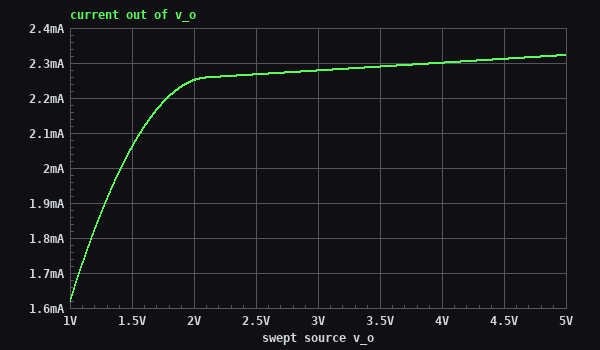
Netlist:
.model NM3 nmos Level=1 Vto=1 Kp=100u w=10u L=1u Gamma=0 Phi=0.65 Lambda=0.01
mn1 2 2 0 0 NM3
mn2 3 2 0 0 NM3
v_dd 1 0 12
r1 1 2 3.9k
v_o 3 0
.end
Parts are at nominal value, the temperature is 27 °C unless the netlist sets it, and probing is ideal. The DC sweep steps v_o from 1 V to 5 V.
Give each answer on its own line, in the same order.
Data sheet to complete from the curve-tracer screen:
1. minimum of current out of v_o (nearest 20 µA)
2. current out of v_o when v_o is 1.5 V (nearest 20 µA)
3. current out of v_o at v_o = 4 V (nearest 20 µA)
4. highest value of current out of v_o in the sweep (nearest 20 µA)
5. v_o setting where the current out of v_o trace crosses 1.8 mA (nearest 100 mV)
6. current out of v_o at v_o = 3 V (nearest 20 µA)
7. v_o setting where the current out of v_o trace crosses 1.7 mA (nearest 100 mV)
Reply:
1.62 mA
2.06 mA
2.30 mA
2.32 mA
1.2 V
2.28 mA
1.1 V
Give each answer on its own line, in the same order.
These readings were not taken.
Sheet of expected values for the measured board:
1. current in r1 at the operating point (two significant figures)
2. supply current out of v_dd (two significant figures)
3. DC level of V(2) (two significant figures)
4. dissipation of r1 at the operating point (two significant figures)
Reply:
2.3 mA
2.3 mA
3.1 V
20 mW
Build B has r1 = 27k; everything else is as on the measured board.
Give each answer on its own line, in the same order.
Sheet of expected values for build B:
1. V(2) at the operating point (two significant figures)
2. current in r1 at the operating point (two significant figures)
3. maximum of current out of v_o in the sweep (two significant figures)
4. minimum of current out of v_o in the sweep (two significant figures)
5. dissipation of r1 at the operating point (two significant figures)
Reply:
1.9 V
380 µA
390 µA
370 µA
3.8 mW
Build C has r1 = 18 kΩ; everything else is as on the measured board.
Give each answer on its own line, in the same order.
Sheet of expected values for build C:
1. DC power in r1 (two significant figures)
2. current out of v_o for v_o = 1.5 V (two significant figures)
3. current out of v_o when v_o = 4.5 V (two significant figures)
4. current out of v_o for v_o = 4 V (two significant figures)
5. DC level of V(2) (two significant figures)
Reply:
5.5 mW
550 µA
570 µA
560 µA
2.0 V
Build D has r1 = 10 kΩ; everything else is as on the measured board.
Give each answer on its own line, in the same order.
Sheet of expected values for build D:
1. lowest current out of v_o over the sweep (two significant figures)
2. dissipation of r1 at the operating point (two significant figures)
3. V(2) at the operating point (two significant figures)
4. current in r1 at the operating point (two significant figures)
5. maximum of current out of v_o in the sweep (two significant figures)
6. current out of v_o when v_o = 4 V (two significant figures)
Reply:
880 µA
9.3 mW
2.4 V
960 µA
990 µA
980 µA
